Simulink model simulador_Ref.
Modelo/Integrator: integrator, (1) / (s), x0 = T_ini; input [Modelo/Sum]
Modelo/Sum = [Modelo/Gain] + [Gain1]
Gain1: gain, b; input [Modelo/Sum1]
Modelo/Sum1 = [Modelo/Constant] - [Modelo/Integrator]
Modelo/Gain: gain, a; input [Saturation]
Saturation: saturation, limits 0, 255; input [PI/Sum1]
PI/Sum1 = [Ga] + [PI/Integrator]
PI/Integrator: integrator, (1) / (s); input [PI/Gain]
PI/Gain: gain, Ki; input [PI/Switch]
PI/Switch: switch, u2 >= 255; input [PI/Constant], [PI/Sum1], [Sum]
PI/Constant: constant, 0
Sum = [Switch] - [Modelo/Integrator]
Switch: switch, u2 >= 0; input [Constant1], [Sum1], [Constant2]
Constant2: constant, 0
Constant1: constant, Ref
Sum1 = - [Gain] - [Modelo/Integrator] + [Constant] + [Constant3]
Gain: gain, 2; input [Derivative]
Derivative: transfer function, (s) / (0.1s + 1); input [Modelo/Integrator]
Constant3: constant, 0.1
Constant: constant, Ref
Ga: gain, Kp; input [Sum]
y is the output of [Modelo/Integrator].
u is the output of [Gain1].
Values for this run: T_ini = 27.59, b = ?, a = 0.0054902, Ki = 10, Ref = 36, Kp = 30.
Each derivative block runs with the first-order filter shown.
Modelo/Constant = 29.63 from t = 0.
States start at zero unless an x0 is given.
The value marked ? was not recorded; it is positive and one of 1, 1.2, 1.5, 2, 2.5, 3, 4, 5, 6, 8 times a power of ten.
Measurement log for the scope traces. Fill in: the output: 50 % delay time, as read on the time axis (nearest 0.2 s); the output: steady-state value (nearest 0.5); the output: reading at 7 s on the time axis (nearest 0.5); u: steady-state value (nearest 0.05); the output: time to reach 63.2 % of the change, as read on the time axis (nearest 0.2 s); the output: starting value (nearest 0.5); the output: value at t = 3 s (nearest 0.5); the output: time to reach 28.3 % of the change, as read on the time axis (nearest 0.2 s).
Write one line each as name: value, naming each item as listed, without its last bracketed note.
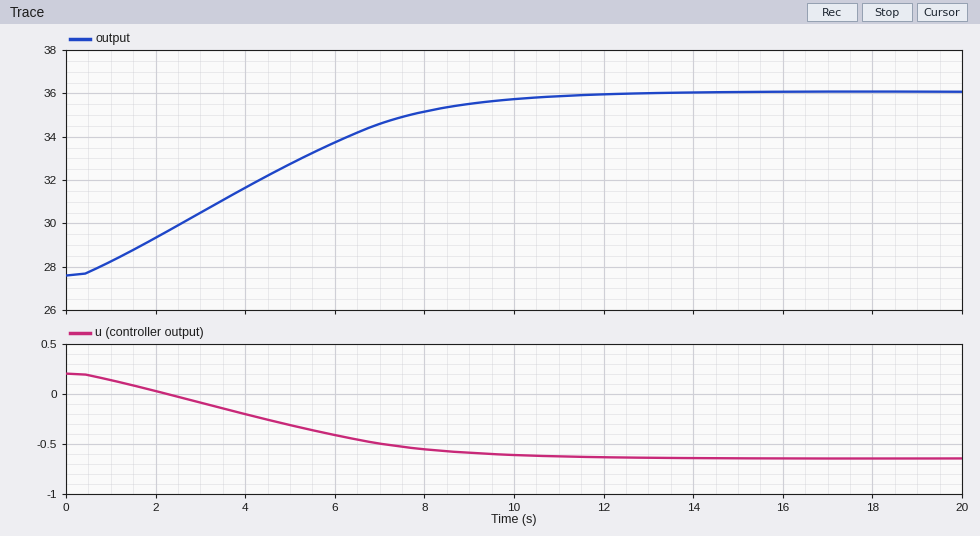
the output: 50 % delay time, as read on the time axis: 4.2 s
the output: steady-state value: 36.0
the output: reading at 7 s on the time axis: 34.5
u: steady-state value: -0.65
the output: time to reach 63.2 % of the change, as read on the time axis: 5.2 s
the output: starting value: 27.5
the output: value at t = 3 s: 30.5
the output: time to reach 28.3 % of the change, as read on the time axis: 2.6 s
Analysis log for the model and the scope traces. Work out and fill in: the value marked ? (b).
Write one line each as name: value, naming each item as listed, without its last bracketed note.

the value marked ?: 0.1
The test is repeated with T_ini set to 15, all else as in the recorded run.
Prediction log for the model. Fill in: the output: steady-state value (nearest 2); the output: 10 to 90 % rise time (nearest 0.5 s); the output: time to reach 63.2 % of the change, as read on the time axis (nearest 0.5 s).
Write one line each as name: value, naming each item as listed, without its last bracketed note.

the output: steady-state value: 36
the output: 10 to 90 % rise time: 10.0 s
the output: time to reach 63.2 % of the change, as read on the time axis: 6.5 s
